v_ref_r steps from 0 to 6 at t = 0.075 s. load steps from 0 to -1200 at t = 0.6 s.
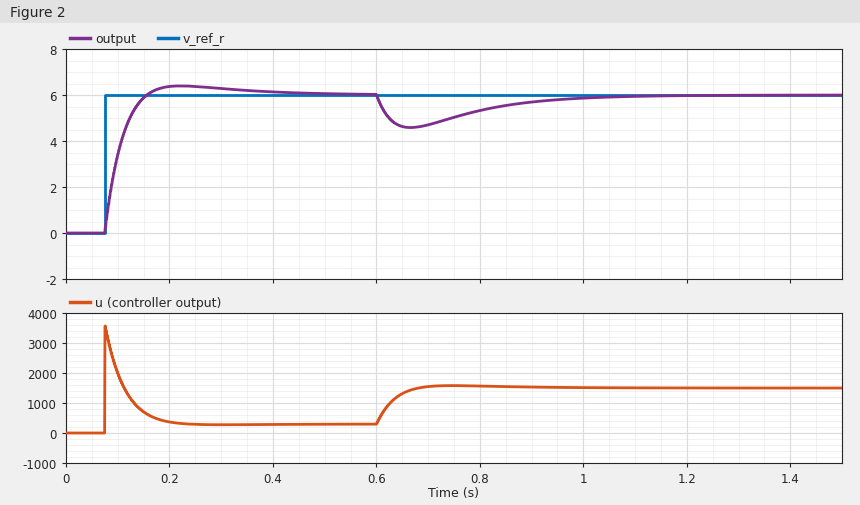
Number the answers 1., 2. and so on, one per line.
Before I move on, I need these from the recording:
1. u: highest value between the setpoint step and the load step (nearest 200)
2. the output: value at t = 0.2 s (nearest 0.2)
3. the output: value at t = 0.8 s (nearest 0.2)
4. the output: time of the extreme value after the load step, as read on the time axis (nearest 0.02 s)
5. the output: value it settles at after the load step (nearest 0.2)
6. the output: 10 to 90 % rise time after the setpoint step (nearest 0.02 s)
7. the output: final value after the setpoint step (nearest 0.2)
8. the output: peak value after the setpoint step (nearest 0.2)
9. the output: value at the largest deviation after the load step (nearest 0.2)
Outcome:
1. 3600
2. 6.4
3. 5.4
4. 0.66 s
5. 6.0
6. 0.06 s
7. 6.0
8. 6.4
9. 4.6
